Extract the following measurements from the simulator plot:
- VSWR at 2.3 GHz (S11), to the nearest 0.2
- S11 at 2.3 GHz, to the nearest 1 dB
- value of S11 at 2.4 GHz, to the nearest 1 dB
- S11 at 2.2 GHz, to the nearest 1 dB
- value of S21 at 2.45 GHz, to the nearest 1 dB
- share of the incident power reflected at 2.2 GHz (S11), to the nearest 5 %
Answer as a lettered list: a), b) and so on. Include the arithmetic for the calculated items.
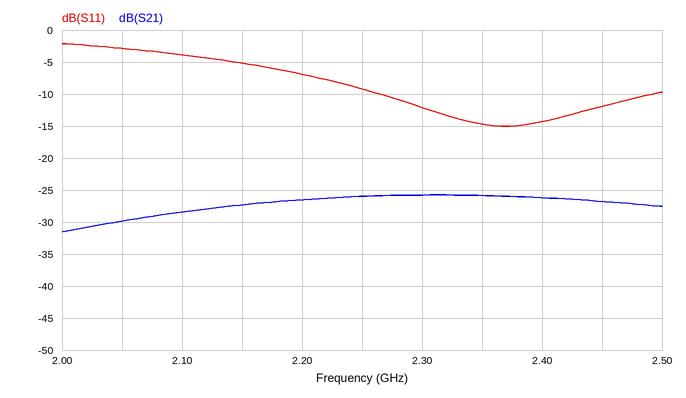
a) |Γ| = 10^(-12/20) = 0.2512; VSWR = (1 + 0.2512)/(1 − 0.2512) ≈ 1.67, so 1.6 to the nearest 0.2
b) -12 dB
c) -14 dB
d) -7 dB
e) -27 dB
f) 10^(-7/10) ≈ 20 %
